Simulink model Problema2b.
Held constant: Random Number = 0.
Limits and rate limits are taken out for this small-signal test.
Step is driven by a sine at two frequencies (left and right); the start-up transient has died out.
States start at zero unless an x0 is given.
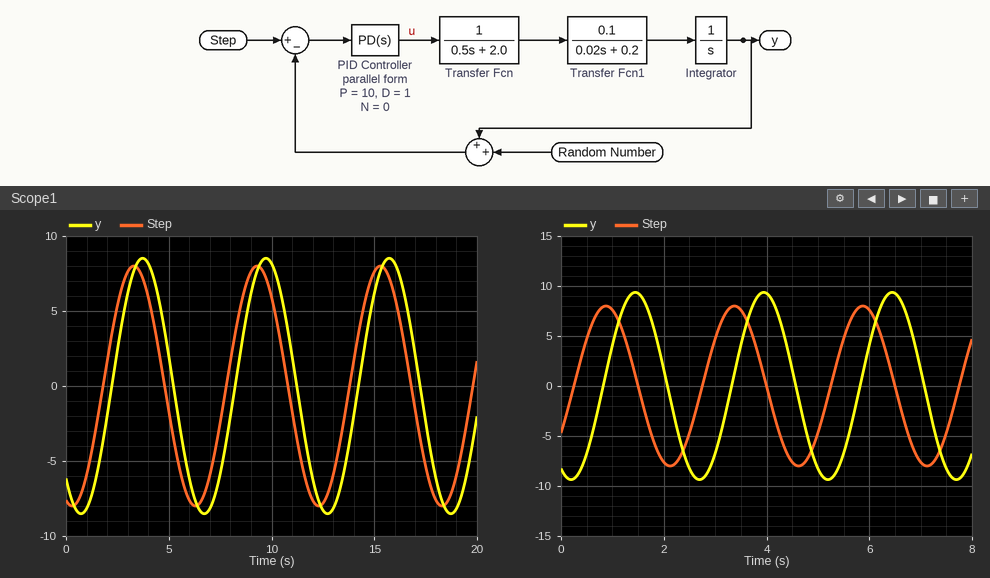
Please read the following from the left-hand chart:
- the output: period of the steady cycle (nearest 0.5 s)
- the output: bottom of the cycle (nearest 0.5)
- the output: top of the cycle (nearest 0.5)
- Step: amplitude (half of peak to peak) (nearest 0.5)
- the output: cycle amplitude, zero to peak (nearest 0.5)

6.0 s
-8.5
8.5
8.0
8.5
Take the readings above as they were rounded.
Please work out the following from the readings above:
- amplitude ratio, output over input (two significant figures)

1.1
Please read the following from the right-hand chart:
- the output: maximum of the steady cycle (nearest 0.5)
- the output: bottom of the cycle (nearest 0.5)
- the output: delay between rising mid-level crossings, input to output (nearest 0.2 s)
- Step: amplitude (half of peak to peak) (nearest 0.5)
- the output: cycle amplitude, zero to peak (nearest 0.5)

9.5
-9.5
0.6 s
8.0
9.5
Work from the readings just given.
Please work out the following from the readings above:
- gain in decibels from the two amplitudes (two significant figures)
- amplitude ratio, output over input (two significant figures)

1.5 dB
1.2
